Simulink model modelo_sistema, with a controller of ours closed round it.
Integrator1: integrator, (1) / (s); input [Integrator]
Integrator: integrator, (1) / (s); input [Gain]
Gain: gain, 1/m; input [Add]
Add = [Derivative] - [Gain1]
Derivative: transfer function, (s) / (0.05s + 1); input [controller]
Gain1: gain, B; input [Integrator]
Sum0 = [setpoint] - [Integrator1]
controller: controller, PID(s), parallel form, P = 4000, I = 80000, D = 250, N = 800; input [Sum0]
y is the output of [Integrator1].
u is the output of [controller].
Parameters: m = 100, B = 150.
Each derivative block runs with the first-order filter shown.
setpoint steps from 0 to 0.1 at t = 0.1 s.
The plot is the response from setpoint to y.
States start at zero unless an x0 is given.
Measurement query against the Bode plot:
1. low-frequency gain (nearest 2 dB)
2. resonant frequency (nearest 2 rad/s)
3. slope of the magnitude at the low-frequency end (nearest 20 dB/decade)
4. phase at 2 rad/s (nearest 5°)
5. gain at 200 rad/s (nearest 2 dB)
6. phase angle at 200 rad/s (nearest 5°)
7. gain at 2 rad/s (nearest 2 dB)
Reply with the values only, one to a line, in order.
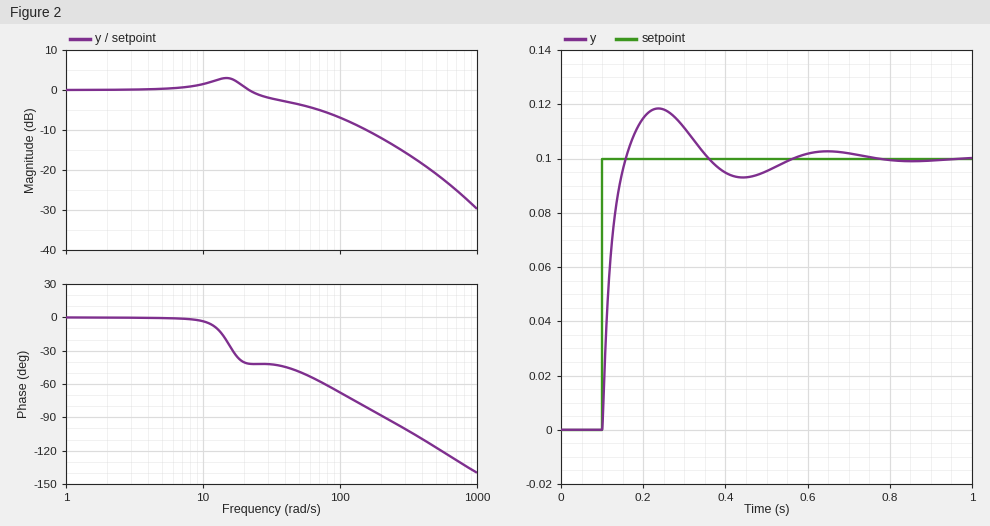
0 dB
14 rad/s
0 dB/decade
0°
-12 dB
-90°
0 dB
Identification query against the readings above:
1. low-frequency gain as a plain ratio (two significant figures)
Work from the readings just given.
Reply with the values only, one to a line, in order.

1.0
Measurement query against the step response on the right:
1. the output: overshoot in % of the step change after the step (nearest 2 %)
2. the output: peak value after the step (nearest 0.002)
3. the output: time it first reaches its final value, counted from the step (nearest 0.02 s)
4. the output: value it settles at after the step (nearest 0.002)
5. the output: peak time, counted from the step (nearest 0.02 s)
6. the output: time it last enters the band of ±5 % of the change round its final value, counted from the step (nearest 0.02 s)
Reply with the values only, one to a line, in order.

18 %
0.118
0.06 s
0.100
0.14 s
0.40 s
